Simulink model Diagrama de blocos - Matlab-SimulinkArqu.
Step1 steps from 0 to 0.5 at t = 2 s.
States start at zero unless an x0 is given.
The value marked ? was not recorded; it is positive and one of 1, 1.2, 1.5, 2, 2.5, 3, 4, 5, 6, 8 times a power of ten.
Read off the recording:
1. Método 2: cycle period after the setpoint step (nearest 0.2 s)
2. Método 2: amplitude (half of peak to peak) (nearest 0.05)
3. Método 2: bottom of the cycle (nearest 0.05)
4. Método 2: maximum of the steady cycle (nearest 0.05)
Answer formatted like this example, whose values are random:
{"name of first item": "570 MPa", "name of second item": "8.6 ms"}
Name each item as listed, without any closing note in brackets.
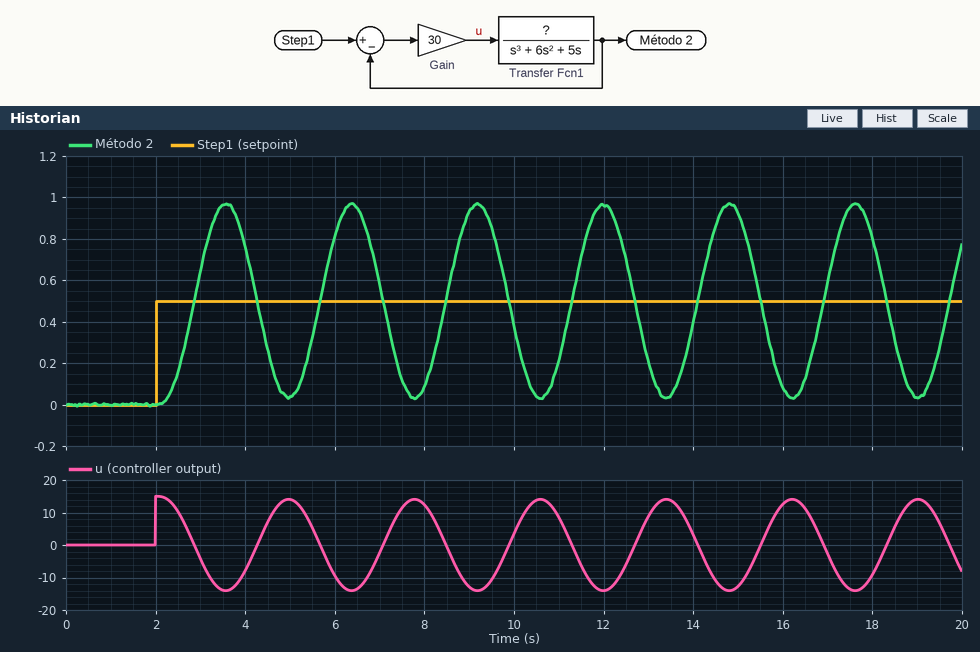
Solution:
{"Método 2: cycle period after the setpoint step": "2.8 s", "Método 2: amplitude (half of peak to peak)": "0.45", "Método 2: bottom of the cycle": "0.05", "Método 2: maximum of the steady cycle": "0.95"}
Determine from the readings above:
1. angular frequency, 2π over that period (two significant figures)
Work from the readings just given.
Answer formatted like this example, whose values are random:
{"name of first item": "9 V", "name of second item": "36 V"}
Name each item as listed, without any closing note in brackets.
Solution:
{"angular frequency, 2π over that period": "2.2 rad/s"}
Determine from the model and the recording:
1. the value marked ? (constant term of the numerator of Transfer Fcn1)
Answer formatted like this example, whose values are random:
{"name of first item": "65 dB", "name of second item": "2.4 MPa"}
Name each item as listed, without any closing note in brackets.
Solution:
{"the value marked ?": "1"}
